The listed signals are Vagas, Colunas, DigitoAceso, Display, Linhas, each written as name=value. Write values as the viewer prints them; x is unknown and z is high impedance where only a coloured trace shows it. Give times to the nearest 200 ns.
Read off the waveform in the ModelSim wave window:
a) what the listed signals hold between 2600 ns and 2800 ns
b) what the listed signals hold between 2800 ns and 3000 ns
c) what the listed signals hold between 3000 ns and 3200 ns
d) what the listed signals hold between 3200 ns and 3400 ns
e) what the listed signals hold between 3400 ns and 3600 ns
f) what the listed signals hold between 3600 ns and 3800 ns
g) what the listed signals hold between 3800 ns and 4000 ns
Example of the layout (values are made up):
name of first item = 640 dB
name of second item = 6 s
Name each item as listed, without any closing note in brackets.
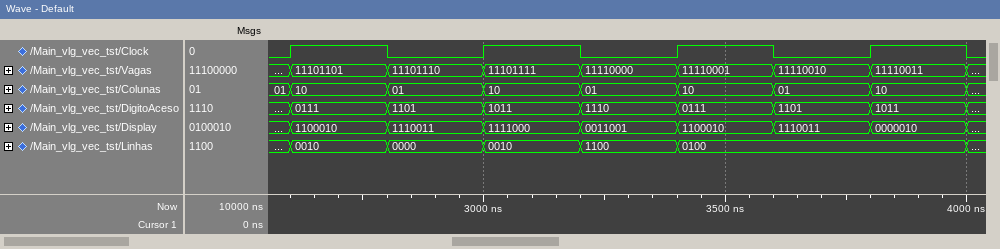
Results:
what the listed signals hold between 2600 ns and 2800 ns = Vagas=11101101, Colunas=10, DigitoAceso=0111, Display=1100010, Linhas=0010
what the listed signals hold between 2800 ns and 3000 ns = Vagas=11101110, Colunas=01, DigitoAceso=1101, Display=1110011, Linhas=0000
what the listed signals hold between 3000 ns and 3200 ns = Vagas=11101111, Colunas=10, DigitoAceso=1011, Display=1111000, Linhas=0010
what the listed signals hold between 3200 ns and 3400 ns = Vagas=11110000, Colunas=01, DigitoAceso=1110, Display=0011001, Linhas=1100
what the listed signals hold between 3400 ns and 3600 ns = Vagas=11110001, Colunas=10, DigitoAceso=0111, Display=1100010, Linhas=0100
what the listed signals hold between 3600 ns and 3800 ns = Vagas=11110010, Colunas=01, DigitoAceso=1101, Display=1110011, Linhas=0100
what the listed signals hold between 3800 ns and 4000 ns = Vagas=11110011, Colunas=10, DigitoAceso=1011, Display=0000010, Linhas=0100
